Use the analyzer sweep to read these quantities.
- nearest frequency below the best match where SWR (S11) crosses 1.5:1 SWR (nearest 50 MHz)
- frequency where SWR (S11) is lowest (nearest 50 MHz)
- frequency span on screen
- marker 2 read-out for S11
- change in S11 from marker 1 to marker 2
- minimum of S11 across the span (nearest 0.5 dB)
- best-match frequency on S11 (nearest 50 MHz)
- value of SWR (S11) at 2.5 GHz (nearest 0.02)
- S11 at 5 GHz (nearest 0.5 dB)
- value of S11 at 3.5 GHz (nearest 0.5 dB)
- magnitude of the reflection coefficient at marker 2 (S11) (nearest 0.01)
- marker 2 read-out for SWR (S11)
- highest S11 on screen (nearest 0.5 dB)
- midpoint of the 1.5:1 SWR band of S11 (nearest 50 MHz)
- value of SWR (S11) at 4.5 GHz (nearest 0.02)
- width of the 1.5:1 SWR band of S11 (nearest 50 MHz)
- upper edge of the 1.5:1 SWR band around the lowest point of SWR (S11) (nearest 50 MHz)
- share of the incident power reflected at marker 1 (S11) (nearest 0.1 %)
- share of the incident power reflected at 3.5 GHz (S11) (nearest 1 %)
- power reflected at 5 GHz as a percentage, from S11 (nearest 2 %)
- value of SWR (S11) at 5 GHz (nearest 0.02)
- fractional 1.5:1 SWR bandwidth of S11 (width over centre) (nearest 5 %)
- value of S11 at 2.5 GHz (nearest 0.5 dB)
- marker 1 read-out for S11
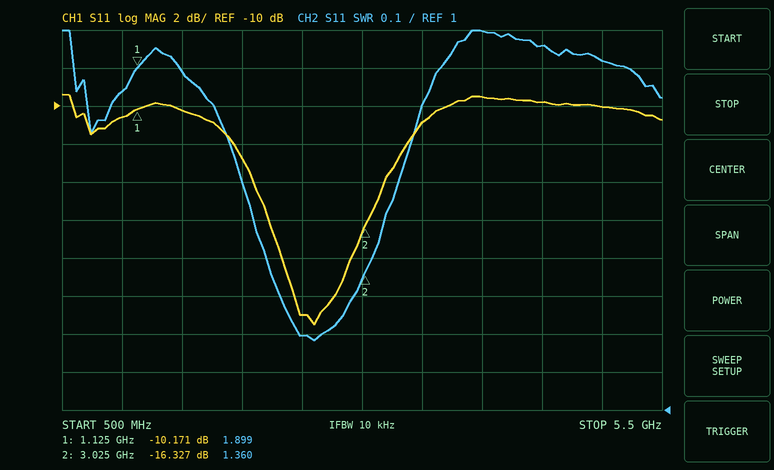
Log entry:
2.10 GHz
2.60 GHz
5 GHz
-16.327 dB
-6.156 dB
-21.5 dB
2.60 GHz
1.20
-10.0 dB
-11.0 dB
0.15
1.360
-9.5 dB
2.65 GHz
1.96
1.10 GHz
3.20 GHz
9.6 %
8 %
10 %
1.92
40 %
-21.0 dB
-10.171 dB
